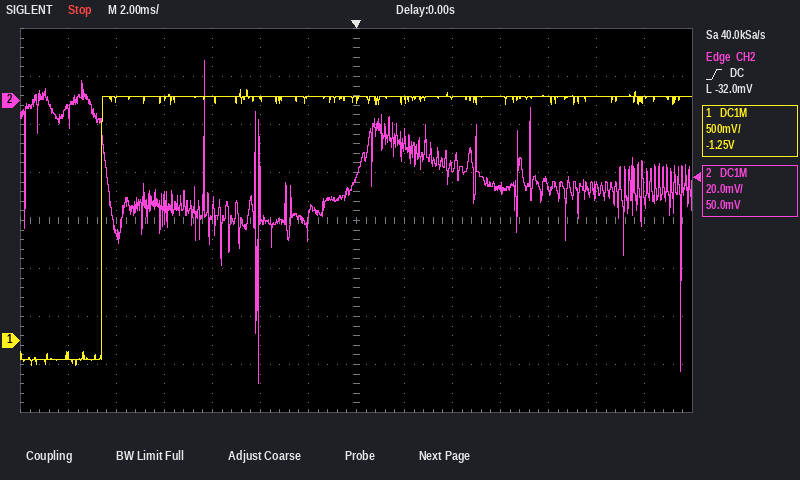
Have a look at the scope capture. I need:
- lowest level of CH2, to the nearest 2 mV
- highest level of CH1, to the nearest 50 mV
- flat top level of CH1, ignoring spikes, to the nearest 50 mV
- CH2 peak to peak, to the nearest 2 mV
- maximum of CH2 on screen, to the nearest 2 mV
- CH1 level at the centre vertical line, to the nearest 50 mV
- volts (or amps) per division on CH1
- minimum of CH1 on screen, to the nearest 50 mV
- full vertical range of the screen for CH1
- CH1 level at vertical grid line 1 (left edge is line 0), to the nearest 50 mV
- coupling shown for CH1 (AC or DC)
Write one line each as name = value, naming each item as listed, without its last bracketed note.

lowest level of CH2, to the nearest 2 mV = -118 mV
highest level of CH1, to the nearest 50 mV = 2.60 V
flat top level of CH1, ignoring spikes, to the nearest 50 mV = 2.55 V
CH2 peak to peak, to the nearest 2 mV = 134 mV
maximum of CH2 on screen, to the nearest 2 mV = 16 mV
CH1 level at the centre vertical line, to the nearest 50 mV = 2.50 V
volts (or amps) per division on CH1 = 500 mV
minimum of CH1 on screen, to the nearest 50 mV = -250 mV
full vertical range of the screen for CH1 = 4 V
CH1 level at vertical grid line 1 (left edge is line 0), to the nearest 50 mV = -150 mV
coupling shown for CH1 = DC
